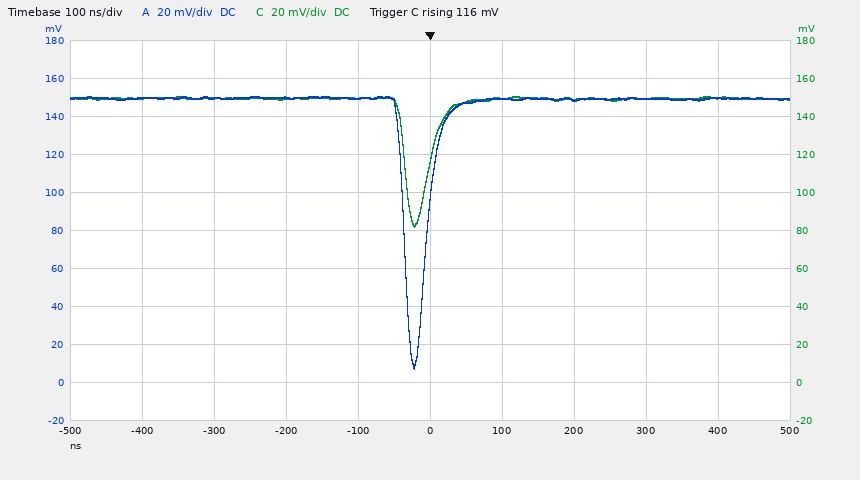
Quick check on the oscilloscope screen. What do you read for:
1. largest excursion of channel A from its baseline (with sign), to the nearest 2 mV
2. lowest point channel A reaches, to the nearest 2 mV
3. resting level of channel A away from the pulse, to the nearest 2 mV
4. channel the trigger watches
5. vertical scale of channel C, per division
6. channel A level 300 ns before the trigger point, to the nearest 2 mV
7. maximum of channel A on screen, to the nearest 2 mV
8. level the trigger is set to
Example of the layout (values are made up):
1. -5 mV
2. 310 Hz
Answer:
1. -142 mV
2. 8 mV
3. 150 mV
4. channel C
5. 20 mV
6. 150 mV
7. 150 mV
8. 116 mV
